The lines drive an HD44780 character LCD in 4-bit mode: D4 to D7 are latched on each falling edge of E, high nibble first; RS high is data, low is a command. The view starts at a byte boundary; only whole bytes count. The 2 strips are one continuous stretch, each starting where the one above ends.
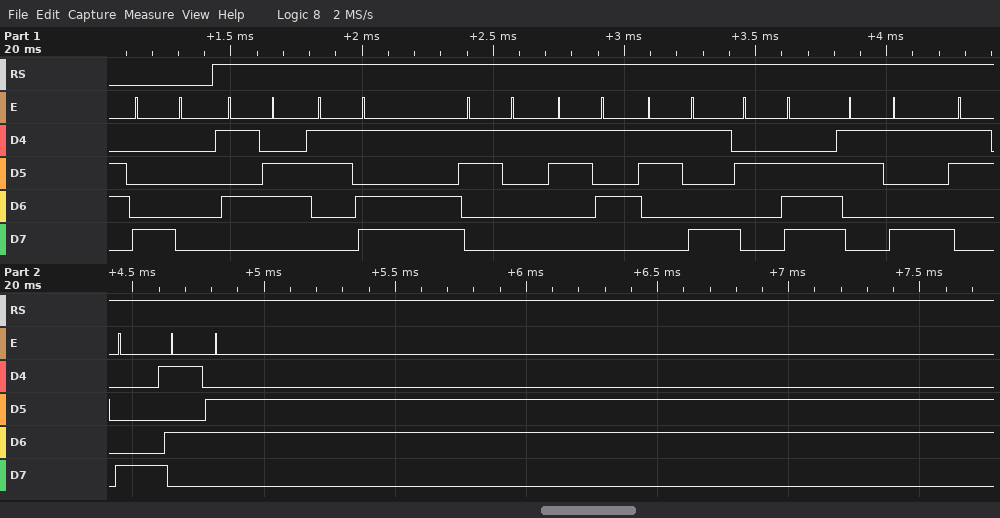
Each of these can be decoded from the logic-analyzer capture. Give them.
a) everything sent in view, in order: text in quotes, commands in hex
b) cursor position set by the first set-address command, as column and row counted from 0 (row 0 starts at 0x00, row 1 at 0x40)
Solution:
0x80 "V=159.98V"
column 0, row 0
